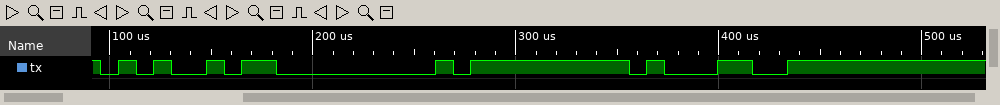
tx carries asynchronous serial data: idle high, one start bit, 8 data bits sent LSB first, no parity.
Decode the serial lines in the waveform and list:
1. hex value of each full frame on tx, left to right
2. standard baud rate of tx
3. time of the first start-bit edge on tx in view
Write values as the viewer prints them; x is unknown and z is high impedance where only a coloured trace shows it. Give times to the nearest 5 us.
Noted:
A5, 00, FF, 31
115200 baud
95 us
